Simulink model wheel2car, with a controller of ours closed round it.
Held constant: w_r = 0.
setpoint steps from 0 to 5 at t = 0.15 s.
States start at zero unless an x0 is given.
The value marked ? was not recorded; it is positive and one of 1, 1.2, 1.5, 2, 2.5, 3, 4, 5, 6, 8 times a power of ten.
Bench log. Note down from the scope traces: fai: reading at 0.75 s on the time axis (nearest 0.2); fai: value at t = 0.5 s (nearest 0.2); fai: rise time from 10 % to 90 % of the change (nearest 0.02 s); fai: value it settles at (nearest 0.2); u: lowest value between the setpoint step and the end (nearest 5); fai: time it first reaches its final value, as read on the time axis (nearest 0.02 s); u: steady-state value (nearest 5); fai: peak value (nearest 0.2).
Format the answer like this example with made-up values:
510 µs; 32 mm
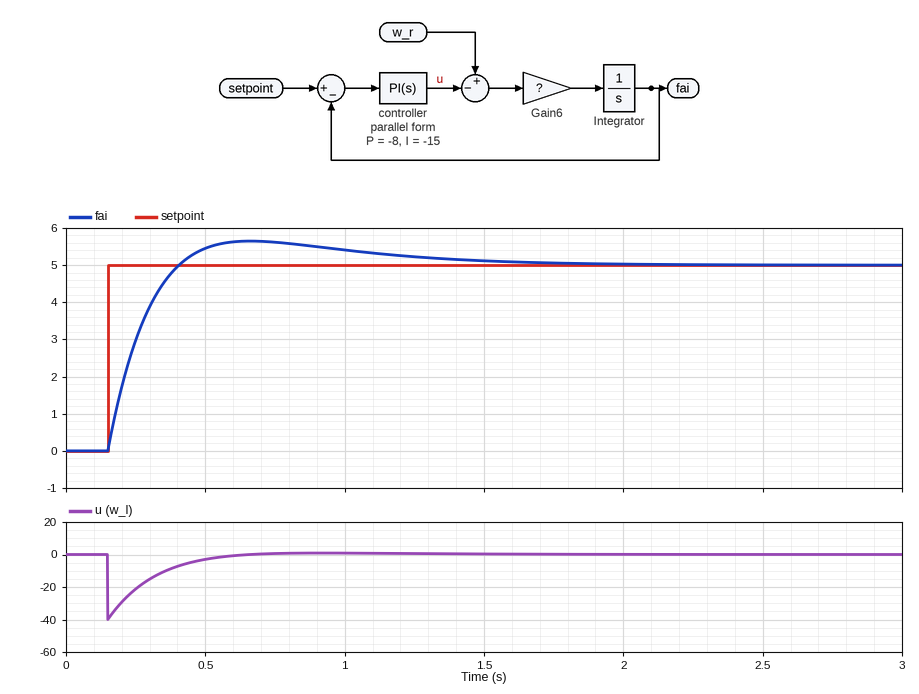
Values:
5.6; 5.4; 0.18 s; 5.0; -40; 0.40 s; 0; 5.6
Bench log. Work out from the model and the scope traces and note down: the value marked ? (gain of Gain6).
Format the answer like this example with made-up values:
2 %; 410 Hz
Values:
1
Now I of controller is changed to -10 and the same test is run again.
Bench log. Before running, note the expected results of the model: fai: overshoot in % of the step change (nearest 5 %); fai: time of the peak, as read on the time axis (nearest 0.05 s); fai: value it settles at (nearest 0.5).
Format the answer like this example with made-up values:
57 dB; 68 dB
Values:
10 %; 0.75 s; 5.0
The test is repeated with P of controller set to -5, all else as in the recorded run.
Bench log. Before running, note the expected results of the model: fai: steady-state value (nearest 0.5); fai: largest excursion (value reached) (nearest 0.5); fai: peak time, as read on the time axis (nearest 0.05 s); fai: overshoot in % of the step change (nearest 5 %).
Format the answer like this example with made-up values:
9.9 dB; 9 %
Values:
5.0; 6.0; 0.75 s; 25 %
